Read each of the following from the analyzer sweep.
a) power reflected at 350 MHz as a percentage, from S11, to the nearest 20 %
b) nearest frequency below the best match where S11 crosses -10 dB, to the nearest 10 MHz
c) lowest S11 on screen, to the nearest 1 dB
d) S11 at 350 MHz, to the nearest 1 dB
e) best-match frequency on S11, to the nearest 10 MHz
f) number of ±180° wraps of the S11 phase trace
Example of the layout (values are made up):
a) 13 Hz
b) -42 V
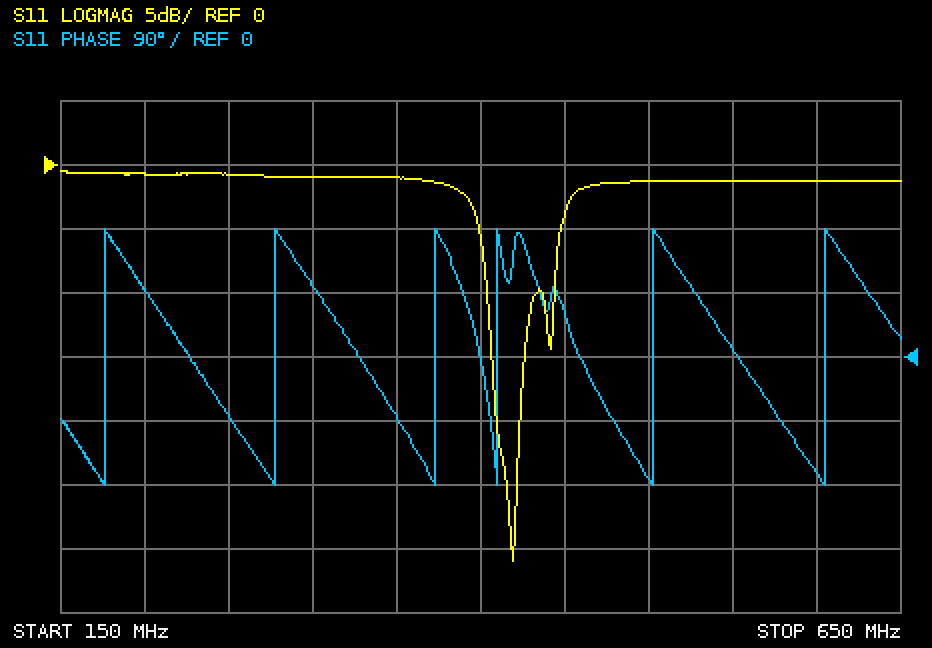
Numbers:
a) 80 %
b) 400 MHz
c) -31 dB
d) -1 dB
e) 420 MHz
f) 6
